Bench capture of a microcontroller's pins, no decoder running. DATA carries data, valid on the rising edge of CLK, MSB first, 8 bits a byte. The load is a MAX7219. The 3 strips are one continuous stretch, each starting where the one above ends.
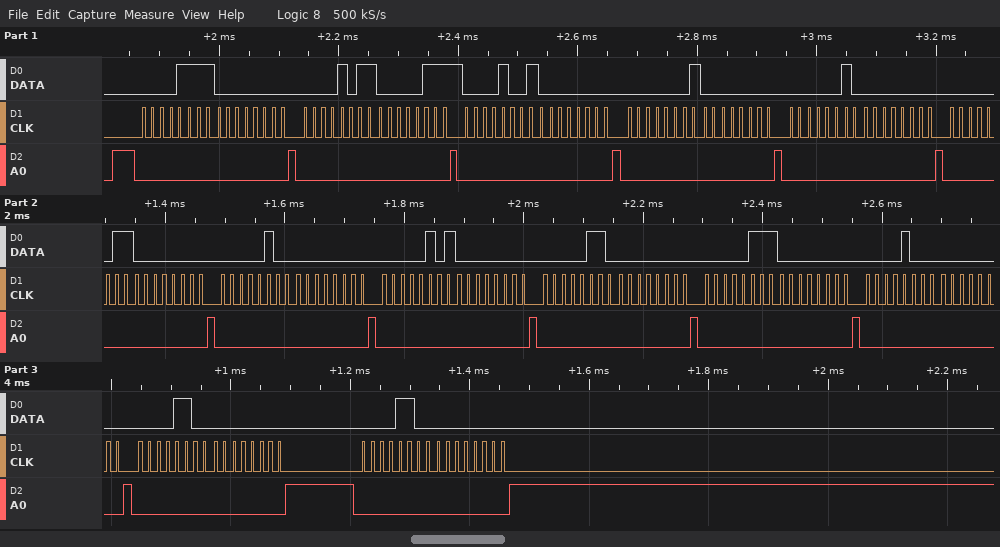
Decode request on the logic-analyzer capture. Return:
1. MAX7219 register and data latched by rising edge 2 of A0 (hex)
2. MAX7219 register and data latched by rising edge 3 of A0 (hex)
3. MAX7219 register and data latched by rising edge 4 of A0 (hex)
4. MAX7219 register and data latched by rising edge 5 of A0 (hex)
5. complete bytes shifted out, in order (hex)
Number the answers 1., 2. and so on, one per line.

1. register 0xF, data 0x00
2. register 0xB, data 0x07
3. register 0x9, data 0x00
4. register 0x1, data 0x00
5. 0x0F 0x00 0x0B 0x07 0x09 0x00 0x01 0x00 0x02 0x00 0x03 0x00 0x04 0x00 0x05 0x00 0x06 0x00 0x07 0x00 0x08 0x00 0x0C 0x00 0x0C 0x00
